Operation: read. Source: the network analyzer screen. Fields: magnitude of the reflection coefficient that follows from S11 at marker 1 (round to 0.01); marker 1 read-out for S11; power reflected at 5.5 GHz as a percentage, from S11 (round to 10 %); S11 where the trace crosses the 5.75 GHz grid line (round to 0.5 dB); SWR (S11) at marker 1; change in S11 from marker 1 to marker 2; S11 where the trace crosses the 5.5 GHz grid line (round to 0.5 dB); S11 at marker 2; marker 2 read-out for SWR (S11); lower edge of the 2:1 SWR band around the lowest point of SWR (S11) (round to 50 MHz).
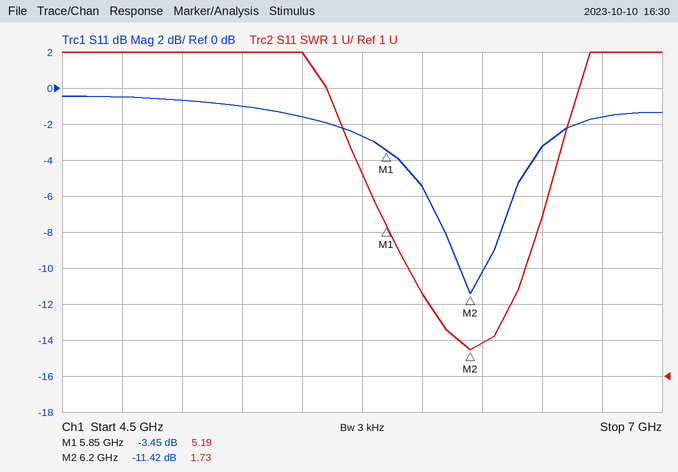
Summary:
0.67
-3.45 dB
70 %
-2.5 dB
5.19
-7.97 dB
-1.5 dB
-11.42 dB
1.73
6.15 GHz
